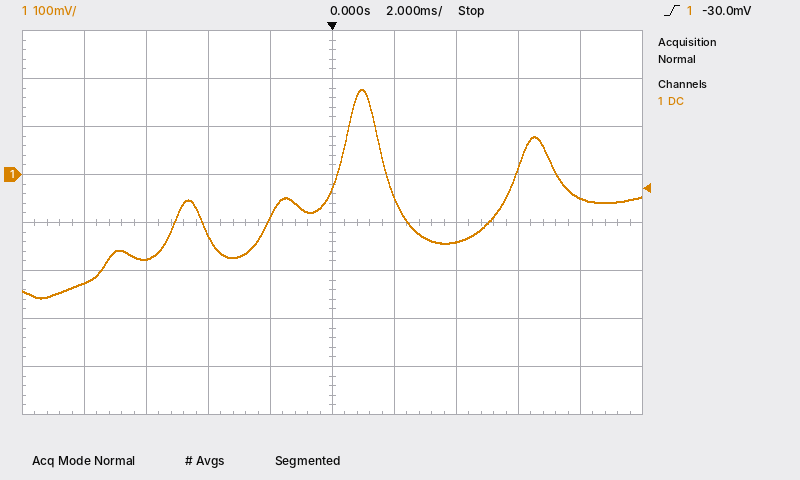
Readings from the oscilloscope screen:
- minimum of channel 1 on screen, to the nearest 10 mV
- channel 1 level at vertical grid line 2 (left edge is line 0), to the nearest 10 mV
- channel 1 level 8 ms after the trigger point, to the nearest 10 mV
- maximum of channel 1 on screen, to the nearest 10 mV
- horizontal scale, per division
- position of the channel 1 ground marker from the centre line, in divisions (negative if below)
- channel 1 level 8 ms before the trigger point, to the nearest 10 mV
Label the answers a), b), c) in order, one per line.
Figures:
a) -260 mV
b) -180 mV
c) -50 mV
d) 180 mV
e) 2 ms
f) +1.0 div
g) -230 mV
